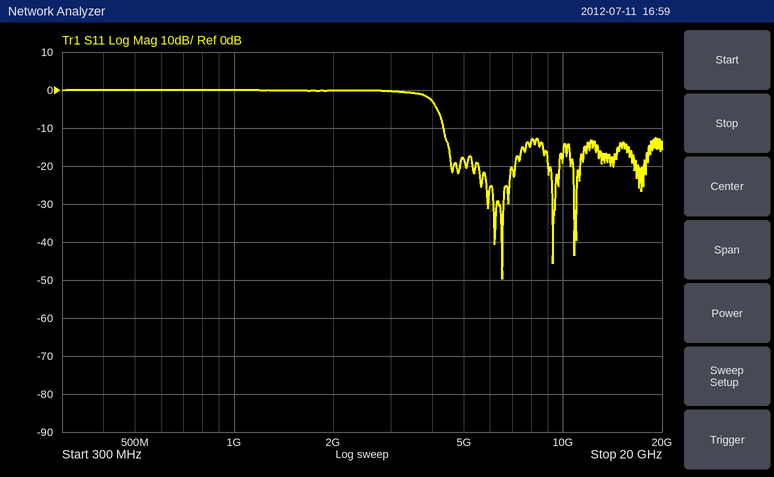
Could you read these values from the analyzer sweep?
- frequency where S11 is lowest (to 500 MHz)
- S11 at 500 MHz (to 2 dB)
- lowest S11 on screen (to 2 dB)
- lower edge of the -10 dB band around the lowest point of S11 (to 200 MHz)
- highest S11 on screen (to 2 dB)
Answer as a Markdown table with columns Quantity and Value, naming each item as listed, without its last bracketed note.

| Quantity | Value |
|---|---|
| frequency where S11 is lowest | 6.5 GHz |
| S11 at 500 MHz | 0 dB |
| lowest S11 on screen | -50 dB |
| lower edge of the -10 dB band around the lowest point of S11 | 4.4 GHz |
| highest S11 on screen | 0 dB |
